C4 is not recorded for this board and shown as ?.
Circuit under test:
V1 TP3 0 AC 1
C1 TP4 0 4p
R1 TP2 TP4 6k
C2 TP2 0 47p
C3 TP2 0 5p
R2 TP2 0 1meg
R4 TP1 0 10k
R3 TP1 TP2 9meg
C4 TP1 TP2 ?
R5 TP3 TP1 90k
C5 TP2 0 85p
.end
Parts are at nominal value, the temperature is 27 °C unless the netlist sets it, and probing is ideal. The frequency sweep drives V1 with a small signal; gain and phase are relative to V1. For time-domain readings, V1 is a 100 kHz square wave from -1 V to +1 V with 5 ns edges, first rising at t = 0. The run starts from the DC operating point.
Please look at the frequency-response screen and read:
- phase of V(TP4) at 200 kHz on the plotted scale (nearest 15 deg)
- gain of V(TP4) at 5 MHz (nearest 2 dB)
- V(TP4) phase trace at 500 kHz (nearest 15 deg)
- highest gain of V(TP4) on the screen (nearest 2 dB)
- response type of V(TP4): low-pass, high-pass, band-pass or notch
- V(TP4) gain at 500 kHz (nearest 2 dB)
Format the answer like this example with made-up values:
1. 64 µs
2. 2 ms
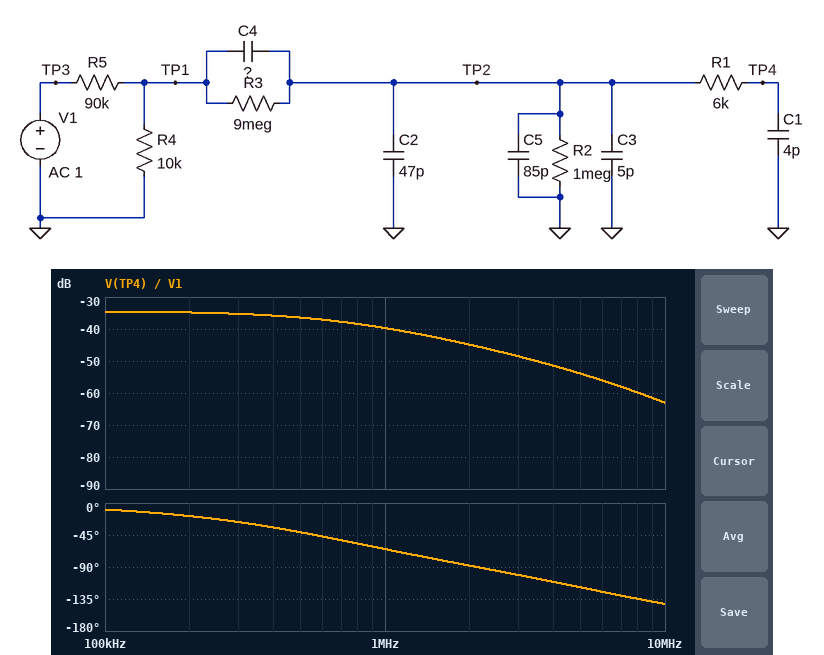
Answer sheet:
1. -15 deg
2. -54 dB
3. -45 deg
4. -34 dB
5. low-pass
6. -36 dB
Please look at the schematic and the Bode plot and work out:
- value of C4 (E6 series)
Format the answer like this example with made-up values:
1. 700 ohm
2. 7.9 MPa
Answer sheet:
1. 33 pF
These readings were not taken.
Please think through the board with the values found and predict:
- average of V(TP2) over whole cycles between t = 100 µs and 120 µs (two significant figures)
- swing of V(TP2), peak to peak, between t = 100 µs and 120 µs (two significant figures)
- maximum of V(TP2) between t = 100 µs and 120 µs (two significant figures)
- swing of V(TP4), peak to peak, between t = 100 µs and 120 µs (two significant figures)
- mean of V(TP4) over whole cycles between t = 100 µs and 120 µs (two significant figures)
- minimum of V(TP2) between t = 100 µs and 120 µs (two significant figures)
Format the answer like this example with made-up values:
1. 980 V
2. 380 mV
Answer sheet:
1. 4.5 mV
2. 38 mV
3. 24 mV
4. 38 mV
5. 4.5 mV
6. -15 mV
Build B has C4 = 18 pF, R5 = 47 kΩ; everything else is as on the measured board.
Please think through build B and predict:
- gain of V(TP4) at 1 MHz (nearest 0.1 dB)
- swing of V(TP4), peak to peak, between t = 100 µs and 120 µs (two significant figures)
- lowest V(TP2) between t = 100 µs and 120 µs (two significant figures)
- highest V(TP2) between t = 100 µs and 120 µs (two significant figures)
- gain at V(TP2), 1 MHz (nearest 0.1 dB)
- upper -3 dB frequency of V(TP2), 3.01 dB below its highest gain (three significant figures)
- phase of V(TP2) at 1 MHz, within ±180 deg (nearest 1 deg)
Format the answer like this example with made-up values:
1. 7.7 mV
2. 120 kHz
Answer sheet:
1. -36.4 dB
2. 40 mV
3. -19 mV
4. 21 mV
5. -36.3 dB
6. 1.21 MHz
7. -39 deg
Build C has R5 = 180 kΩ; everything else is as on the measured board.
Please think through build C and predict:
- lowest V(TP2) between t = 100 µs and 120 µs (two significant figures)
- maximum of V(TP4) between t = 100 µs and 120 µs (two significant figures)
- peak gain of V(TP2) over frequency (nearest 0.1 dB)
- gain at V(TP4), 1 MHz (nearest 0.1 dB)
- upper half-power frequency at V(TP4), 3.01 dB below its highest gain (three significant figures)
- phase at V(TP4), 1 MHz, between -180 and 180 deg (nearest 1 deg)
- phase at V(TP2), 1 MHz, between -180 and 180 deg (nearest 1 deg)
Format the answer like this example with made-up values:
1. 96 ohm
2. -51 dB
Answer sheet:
1. -7.8 mV
2. 12 mV
3. -40.0 dB
4. -45.6 dB
5. 625 kHz
6. -66 deg
7. -58 deg
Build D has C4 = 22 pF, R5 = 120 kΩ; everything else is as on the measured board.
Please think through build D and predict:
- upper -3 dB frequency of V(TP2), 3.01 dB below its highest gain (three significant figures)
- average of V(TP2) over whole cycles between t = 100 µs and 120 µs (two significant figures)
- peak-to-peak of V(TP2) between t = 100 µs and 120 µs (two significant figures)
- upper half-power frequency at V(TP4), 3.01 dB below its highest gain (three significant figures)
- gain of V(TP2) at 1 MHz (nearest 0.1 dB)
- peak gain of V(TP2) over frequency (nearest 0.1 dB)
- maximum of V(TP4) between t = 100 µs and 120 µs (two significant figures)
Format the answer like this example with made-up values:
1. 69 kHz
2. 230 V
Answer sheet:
1. 909 kHz
2. 1.3 mV
3. 21 mV
4. 892 kHz
5. -43.1 dB
6. -39.7 dB
7. 12 mV
